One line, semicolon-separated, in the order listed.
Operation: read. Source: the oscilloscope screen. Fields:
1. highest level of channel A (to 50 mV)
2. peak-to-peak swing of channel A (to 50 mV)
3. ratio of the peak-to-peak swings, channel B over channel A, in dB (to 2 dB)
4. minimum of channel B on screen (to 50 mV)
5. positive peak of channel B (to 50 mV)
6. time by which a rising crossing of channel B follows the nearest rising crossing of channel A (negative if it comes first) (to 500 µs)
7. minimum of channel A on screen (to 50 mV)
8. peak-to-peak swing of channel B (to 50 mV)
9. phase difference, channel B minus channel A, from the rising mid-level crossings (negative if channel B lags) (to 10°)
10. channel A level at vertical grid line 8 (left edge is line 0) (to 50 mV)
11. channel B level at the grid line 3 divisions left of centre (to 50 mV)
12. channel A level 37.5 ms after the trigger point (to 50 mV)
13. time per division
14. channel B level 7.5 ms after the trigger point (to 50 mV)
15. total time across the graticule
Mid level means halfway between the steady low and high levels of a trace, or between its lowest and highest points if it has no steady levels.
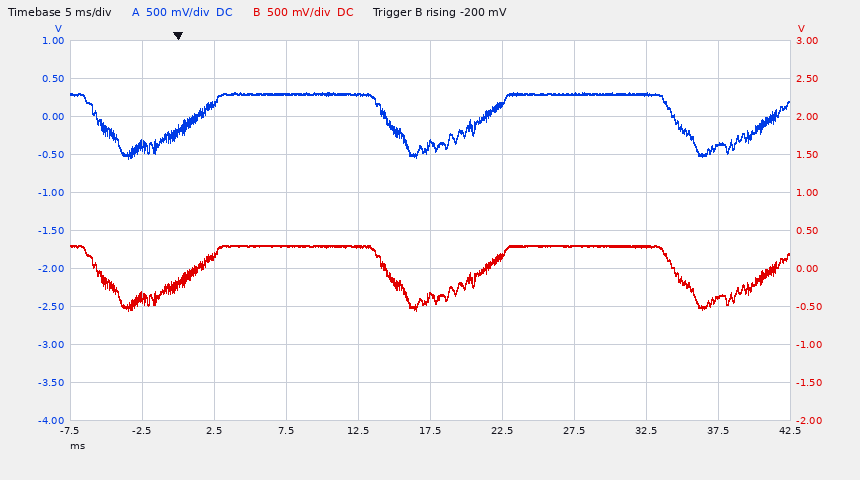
300 mV; 850 mV; 0 dB; -550 mV; 300 mV; 0.0 ms; -550 mV; 850 mV; 0°; 300 mV; 150 mV; -400 mV; 5 ms; 300 mV; 50 ms
